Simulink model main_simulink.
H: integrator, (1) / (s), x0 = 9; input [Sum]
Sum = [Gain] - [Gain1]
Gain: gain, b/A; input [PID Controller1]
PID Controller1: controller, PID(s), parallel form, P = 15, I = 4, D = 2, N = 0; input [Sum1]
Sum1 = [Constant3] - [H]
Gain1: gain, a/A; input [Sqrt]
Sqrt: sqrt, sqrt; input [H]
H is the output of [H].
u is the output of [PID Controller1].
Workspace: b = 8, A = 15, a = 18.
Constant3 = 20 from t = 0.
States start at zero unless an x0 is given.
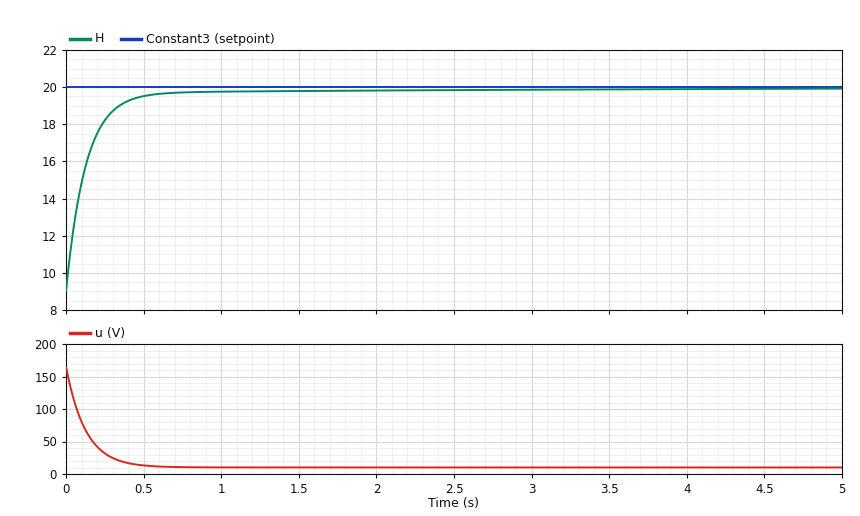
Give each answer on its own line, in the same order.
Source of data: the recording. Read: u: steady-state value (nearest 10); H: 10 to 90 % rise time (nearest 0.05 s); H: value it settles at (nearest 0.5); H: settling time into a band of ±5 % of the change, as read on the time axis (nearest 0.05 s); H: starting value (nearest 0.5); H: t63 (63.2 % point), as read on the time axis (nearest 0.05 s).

10
0.30 s
20.0
0.45 s
9.0
0.15 s
